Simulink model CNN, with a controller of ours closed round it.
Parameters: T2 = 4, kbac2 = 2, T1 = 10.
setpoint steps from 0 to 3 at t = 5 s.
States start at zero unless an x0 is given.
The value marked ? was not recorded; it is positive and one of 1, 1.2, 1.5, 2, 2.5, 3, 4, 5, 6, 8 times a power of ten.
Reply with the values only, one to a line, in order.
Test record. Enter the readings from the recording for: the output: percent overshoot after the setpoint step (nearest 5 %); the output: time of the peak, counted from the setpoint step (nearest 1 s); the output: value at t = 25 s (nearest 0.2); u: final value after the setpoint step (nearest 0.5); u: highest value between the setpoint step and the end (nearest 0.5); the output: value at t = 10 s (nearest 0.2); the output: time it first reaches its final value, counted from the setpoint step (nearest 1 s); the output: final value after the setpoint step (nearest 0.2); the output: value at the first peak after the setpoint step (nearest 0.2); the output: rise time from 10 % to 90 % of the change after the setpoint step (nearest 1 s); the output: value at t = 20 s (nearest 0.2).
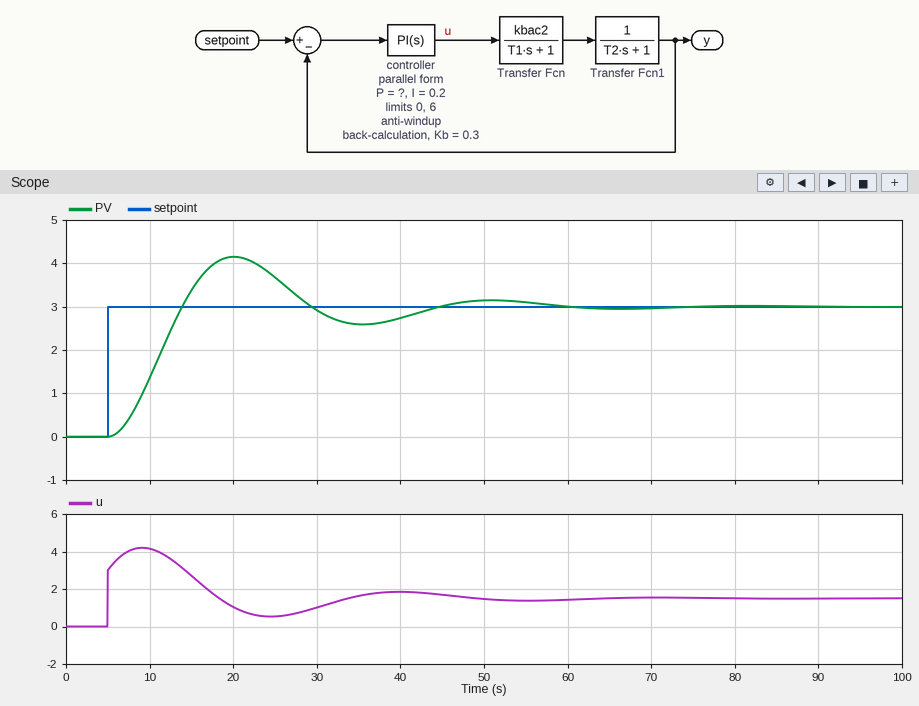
40 %
15 s
3.6
1.5
4.0
1.4
9 s
3.0
4.2
6 s
4.2
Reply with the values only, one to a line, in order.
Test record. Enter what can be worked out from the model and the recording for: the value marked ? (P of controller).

1
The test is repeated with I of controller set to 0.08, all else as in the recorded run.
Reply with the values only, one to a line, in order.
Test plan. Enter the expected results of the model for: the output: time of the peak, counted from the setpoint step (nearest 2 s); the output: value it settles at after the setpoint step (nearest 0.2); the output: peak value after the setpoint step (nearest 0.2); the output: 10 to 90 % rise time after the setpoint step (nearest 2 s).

18 s
3.0
3.2
8 s
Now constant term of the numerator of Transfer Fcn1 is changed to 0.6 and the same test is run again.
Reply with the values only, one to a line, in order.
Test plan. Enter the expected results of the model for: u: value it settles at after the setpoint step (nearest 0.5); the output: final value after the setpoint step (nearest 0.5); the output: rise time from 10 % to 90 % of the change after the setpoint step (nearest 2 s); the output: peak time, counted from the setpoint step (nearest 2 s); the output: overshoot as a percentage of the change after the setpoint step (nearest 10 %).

2.5
3.0
8 s
20 s
30 %
